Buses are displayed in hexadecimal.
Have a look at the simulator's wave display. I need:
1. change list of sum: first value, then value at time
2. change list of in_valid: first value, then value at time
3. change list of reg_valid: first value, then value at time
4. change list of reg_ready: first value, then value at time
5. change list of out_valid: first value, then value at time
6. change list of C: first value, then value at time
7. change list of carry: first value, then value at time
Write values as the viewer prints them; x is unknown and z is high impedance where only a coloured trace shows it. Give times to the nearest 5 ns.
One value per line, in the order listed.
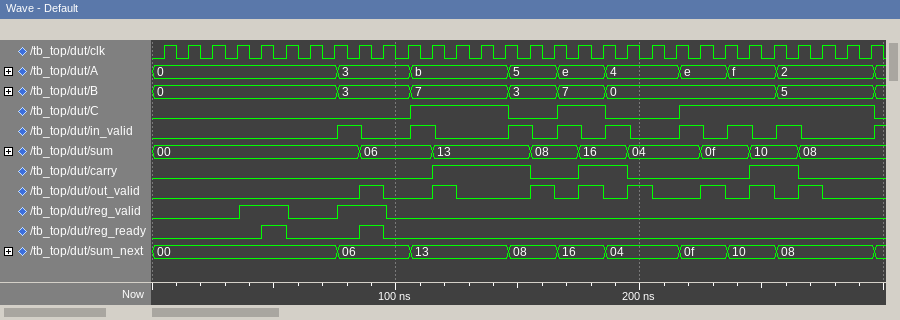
00, 06 at 85 ns, 13 at 115 ns, 08 at 155 ns, 16 at 175 ns, 04 at 195 ns, 0f at 225 ns, 10 at 245 ns, 08 at 265 ns
0, 1 at 75 ns, 0 at 85 ns, 1 at 105 ns, 0 at 115 ns, 1 at 145 ns, 0 at 155 ns, 1 at 165 ns, 0 at 175 ns, 1 at 185 ns, 0 at 195 ns, 1 at 215 ns, 0 at 225 ns, 1 at 235 ns, 0 at 245 ns, 1 at 255 ns, 0 at 265 ns, 1 at 295 ns
0, 1 at 35 ns, 0 at 55 ns, 1 at 75 ns, 0 at 95 ns
0, 1 at 45 ns, 0 at 55 ns, 1 at 85 ns, 0 at 95 ns
0, 1 at 85 ns, 0 at 95 ns, 1 at 115 ns, 0 at 125 ns, 1 at 155 ns, 0 at 165 ns, 1 at 175 ns, 0 at 185 ns, 1 at 195 ns, 0 at 205 ns, 1 at 225 ns, 0 at 235 ns, 1 at 245 ns, 0 at 255 ns, 1 at 265 ns, 0 at 275 ns
0, 1 at 105 ns, 0 at 145 ns, 1 at 165 ns, 0 at 185 ns, 1 at 215 ns, 0 at 295 ns
0, 1 at 115 ns, 0 at 155 ns, 1 at 175 ns, 0 at 195 ns, 1 at 245 ns, 0 at 265 ns
